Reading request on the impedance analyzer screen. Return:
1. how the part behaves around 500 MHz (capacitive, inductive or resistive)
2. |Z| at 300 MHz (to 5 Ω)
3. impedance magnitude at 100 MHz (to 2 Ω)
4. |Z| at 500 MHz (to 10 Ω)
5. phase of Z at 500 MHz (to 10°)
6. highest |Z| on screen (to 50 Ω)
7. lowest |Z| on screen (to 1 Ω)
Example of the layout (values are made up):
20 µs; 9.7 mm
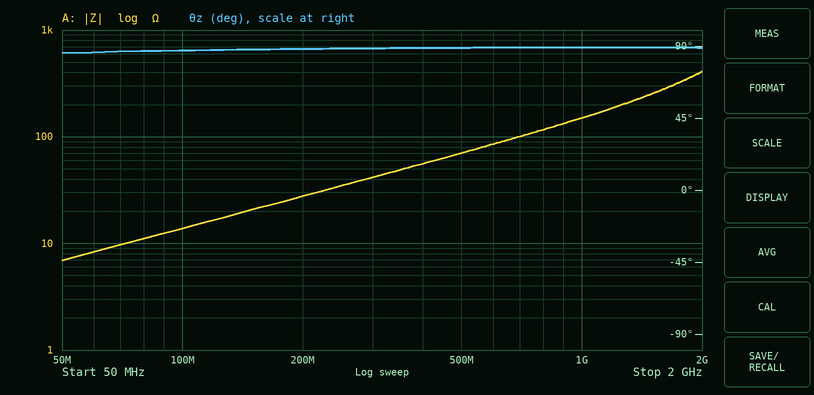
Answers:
inductive; 40 Ω; 14 Ω; 70 Ω; 90°; 400 Ω; 7 Ω
